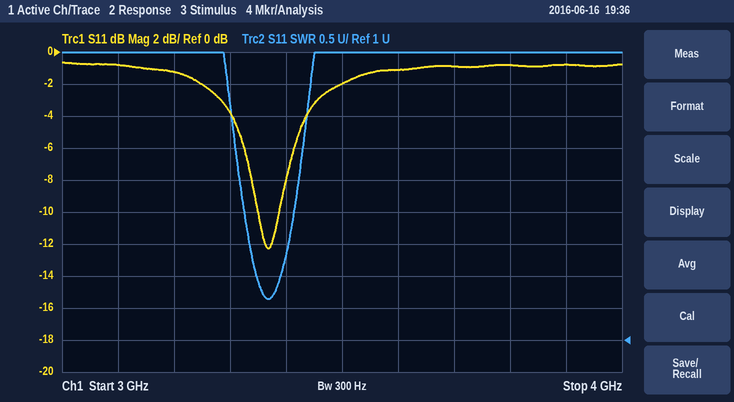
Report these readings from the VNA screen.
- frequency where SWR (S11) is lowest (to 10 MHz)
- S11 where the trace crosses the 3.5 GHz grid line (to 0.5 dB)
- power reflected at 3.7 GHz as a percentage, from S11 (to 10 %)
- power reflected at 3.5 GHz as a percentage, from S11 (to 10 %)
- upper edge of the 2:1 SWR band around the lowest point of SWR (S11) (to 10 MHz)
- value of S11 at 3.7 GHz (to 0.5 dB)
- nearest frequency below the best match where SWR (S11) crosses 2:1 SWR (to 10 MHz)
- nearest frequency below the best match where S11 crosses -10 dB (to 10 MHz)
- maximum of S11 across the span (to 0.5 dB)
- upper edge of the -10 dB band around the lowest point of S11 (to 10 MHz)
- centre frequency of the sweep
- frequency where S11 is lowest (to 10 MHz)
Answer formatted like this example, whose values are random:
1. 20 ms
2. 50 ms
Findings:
1. 3.37 GHz
2. -2.0 dB
3. 80 %
4. 60 %
5. 3.39 GHz
6. -1.0 dB
7. 3.35 GHz
8. 3.35 GHz
9. -0.5 dB
10. 3.39 GHz
11. 3.5 GHz
12. 3.37 GHz
